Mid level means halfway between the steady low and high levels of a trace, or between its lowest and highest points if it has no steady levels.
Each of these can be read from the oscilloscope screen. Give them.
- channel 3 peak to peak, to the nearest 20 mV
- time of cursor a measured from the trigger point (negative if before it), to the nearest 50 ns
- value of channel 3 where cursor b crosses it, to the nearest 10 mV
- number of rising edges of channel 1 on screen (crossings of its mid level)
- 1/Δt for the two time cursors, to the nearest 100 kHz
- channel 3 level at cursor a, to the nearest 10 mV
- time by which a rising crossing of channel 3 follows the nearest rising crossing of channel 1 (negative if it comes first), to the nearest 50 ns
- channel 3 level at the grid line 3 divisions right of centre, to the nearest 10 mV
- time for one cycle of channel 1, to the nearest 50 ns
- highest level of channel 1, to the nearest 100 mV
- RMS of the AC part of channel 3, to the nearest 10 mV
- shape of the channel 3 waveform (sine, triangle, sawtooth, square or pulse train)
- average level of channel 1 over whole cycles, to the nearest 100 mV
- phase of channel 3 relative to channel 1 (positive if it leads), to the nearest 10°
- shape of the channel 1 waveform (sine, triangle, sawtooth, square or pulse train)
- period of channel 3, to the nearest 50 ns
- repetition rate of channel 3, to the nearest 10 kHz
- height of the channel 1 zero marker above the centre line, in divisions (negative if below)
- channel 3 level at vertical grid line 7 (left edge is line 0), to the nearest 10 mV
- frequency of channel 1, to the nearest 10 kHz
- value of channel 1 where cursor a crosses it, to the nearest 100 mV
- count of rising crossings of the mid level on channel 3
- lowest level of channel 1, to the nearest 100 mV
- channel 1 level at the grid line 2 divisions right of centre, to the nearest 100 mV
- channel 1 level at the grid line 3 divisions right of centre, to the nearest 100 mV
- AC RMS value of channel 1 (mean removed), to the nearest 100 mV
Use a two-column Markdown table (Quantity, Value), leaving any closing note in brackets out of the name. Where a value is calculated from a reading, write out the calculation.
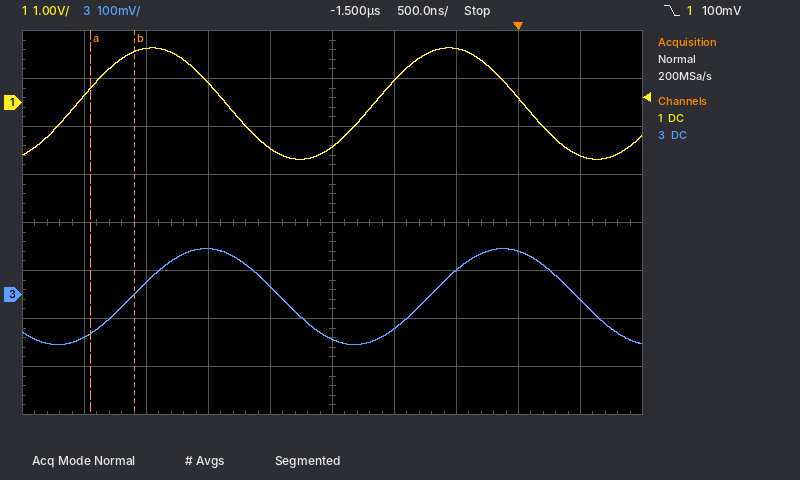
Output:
| Quantity | Value |
|---|---|
| channel 3 peak to peak, to the nearest 20 mV | 200 mV |
| time of cursor a measured from the trigger point (negative if before it), to the nearest 50 ns | -3.45 µs |
| value of channel 3 where cursor b crosses it, to the nearest 10 mV | 0 mV |
| number of rising edges of channel 1 on screen | 2 |
| 1/Δt for the two time cursors, to the nearest 100 kHz | 1 / 350 ns ≈ 2.9 MHz |
| channel 3 level at cursor a, to the nearest 10 mV | -80 mV |
| time by which a rising crossing of channel 3 follows the nearest rising crossing of channel 1 (negative if it comes first), to the nearest 50 ns | +450 ns |
| channel 3 level at the grid line 3 divisions right of centre, to the nearest 10 mV | 90 mV |
| time for one cycle of channel 1, to the nearest 50 ns | 2.40 µs |
| highest level of channel 1, to the nearest 100 mV | 1.1 V |
| RMS of the AC part of channel 3, to the nearest 10 mV | 200 mV / (2√2) ≈ 70.7 mV, so 70 mV to the nearest 10 mV |
| shape of the channel 3 waveform | sine |
| average level of channel 1 over whole cycles, to the nearest 100 mV | (1.1 V + (-1.2 V)) / 2 ≈ 0.0 V |
| phase of channel 3 relative to channel 1 (positive if it leads), to the nearest 10° | −360° × (+450 ns) / 2.40 µs ≈ -67.5°, so -70° to the nearest 10° |
| shape of the channel 1 waveform | sine |
| period of channel 3, to the nearest 50 ns | 2.40 µs |
| repetition rate of channel 3, to the nearest 10 kHz | 1 / 2.40 µs ≈ 417 kHz, so 420 kHz to the nearest 10 kHz |
| height of the channel 1 zero marker above the centre line, in divisions | +2.5 div |
| channel 3 level at vertical grid line 7 (left edge is line 0), to the nearest 10 mV | 50 mV |
| frequency of channel 1, to the nearest 10 kHz | 1 / 2.40 µs ≈ 417 kHz, so 420 kHz to the nearest 10 kHz |
| value of channel 1 where cursor a crosses it, to the nearest 100 mV | 300 mV |
| count of rising crossings of the mid level on channel 3 | 2 |
| lowest level of channel 1, to the nearest 100 mV | -1.2 V |
| channel 1 level at the grid line 2 divisions right of centre, to the nearest 100 mV | 1.1 V |
| channel 1 level at the grid line 3 divisions right of centre, to the nearest 100 mV | 100 mV |
| AC RMS value of channel 1 (mean removed), to the nearest 100 mV | 2.3 V / (2√2) ≈ 813 mV, so 800 mV to the nearest 100 mV |
